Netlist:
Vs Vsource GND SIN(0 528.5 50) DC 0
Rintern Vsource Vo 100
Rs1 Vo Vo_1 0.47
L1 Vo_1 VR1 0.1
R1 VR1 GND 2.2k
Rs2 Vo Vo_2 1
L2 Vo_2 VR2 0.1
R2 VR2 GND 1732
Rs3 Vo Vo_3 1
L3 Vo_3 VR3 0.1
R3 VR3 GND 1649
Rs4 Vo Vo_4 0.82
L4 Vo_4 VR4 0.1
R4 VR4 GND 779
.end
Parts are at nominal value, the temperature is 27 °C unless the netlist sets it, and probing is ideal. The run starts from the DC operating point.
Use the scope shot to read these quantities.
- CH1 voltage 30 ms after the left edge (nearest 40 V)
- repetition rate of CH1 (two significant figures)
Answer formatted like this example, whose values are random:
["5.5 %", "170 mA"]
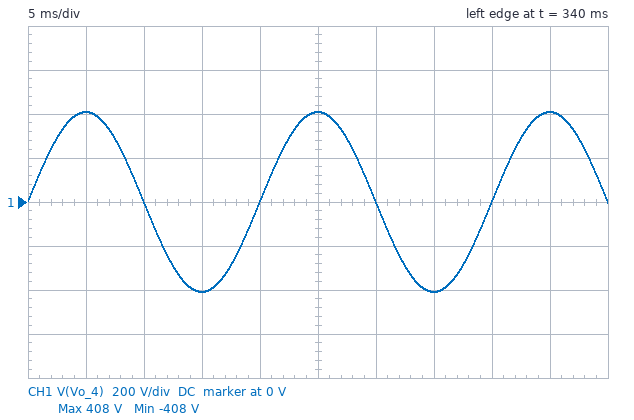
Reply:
["0 V", "50 Hz"]
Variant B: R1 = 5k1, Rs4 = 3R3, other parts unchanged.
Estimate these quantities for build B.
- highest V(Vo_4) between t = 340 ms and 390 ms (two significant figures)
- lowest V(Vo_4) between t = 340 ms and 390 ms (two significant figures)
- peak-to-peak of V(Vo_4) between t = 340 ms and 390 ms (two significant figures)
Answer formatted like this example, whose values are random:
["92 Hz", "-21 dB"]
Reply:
["420 V", "-420 V", "830 V"]
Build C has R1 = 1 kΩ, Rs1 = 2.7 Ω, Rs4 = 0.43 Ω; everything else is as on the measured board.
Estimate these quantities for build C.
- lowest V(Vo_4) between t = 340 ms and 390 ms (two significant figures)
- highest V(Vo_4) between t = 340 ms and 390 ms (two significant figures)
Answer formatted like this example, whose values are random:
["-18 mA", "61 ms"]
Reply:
["-390 V", "390 V"]
